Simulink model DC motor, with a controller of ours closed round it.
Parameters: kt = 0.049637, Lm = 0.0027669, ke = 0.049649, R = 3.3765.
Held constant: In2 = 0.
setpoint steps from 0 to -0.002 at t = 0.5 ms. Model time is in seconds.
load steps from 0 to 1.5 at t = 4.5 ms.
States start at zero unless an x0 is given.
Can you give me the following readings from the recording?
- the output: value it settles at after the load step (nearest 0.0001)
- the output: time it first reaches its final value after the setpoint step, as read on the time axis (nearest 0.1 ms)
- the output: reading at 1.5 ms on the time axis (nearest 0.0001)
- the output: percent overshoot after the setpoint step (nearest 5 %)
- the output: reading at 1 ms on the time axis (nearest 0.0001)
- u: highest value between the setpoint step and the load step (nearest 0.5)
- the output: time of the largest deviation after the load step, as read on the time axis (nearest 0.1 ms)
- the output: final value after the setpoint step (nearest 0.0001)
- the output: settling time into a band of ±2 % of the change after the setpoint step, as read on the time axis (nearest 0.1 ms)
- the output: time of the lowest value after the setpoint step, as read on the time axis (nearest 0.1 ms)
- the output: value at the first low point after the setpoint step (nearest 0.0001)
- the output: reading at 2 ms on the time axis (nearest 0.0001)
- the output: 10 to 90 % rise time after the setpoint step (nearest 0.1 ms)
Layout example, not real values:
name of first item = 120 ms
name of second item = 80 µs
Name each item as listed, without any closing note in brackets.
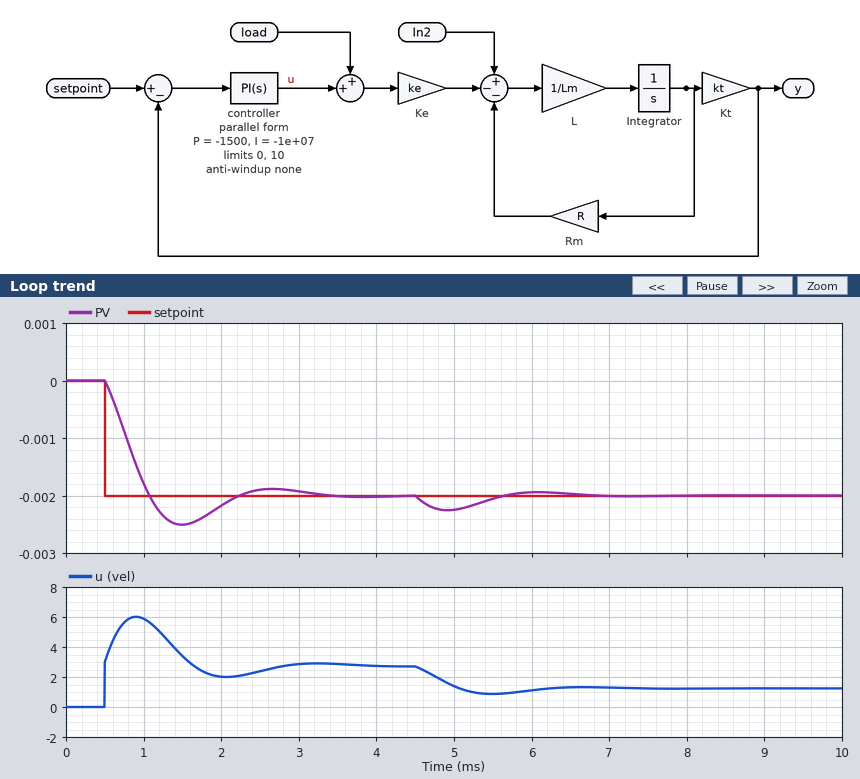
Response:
the output: value it settles at after the load step = -0.0020
the output: time it first reaches its final value after the setpoint step, as read on the time axis = 1.1 ms
the output: reading at 1.5 ms on the time axis = -0.0025
the output: percent overshoot after the setpoint step = 25 %
the output: reading at 1 ms on the time axis = -0.0018
u: highest value between the setpoint step and the load step = 6.0
the output: time of the largest deviation after the load step, as read on the time axis = 4.9 ms
the output: final value after the setpoint step = -0.0020
the output: settling time into a band of ±2 % of the change after the setpoint step, as read on the time axis = 3.2 ms
the output: time of the lowest value after the setpoint step, as read on the time axis = 1.5 ms
the output: value at the first low point after the setpoint step = -0.0025
the output: reading at 2 ms on the time axis = -0.0022
the output: 10 to 90 % rise time after the setpoint step = 0.4 ms
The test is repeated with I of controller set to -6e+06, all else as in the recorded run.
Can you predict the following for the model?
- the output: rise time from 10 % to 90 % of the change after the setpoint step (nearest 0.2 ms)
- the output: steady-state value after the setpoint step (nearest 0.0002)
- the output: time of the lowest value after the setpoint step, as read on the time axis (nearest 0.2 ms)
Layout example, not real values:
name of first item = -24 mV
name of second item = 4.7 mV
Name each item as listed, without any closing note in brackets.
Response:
the output: rise time from 10 % to 90 % of the change after the setpoint step = 0.6 ms
the output: steady-state value after the setpoint step = -0.0020
the output: time of the lowest value after the setpoint step, as read on the time axis = 1.8 ms
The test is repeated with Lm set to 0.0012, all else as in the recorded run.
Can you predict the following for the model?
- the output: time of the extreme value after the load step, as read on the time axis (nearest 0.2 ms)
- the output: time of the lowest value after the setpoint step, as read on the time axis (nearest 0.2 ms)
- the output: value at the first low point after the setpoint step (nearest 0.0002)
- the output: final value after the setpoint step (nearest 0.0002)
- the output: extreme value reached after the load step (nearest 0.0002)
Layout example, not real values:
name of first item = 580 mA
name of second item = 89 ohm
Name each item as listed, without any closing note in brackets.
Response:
the output: time of the extreme value after the load step, as read on the time axis = 4.8 ms
the output: time of the lowest value after the setpoint step, as read on the time axis = 1.2 ms
the output: value at the first low point after the setpoint step = -0.0022
the output: final value after the setpoint step = -0.0020
the output: extreme value reached after the load step = -0.0024
